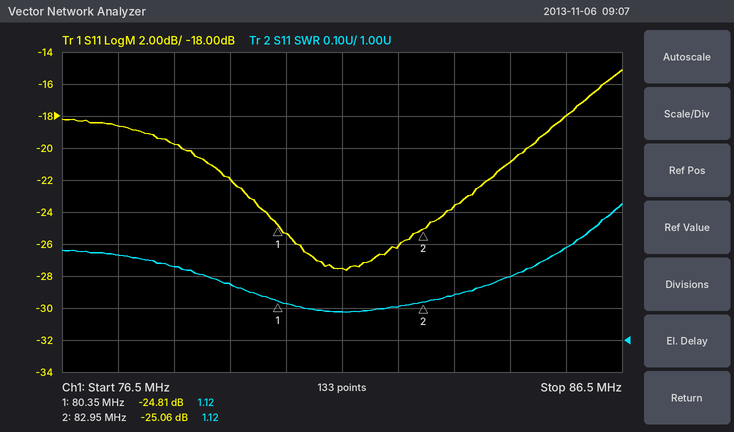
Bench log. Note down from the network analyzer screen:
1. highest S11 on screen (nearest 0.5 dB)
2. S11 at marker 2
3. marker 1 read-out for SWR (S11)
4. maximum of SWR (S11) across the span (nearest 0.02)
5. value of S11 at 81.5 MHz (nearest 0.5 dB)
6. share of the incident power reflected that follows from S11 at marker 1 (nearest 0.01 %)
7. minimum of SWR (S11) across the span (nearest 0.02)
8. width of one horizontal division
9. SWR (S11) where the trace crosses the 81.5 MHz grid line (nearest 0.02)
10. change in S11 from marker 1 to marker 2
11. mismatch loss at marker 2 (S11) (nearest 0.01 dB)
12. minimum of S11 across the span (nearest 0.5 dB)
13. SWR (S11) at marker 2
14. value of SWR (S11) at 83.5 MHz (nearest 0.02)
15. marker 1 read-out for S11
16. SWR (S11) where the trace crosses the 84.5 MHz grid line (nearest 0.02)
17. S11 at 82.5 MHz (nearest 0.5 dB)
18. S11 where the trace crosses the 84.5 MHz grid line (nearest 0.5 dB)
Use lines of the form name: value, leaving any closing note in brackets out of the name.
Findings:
highest S11 on screen: -15.0 dB
S11 at marker 2: -25.06 dB
marker 1 read-out for SWR: 1.12
maximum of SWR (S11) across the span: 1.42
value of S11 at 81.5 MHz: -27.5 dB
share of the incident power reflected that follows from S11 at marker 1: 0.33 %
minimum of SWR (S11) across the span: 1.08
width of one horizontal division: 1 MHz
SWR (S11) where the trace crosses the 81.5 MHz grid line: 1.08
change in S11 from marker 1 to marker 2: -0.25 dB
mismatch loss at marker 2 (S11): 0.01 dB
minimum of S11 across the span: -27.5 dB
SWR (S11) at marker 2: 1.12
value of SWR (S11) at 83.5 MHz: 1.14
marker 1 read-out for S11: -24.81 dB
SWR (S11) where the trace crosses the 84.5 MHz grid line: 1.20
S11 at 82.5 MHz: -26.0 dB
S11 where the trace crosses the 84.5 MHz grid line: -21.0 dB
